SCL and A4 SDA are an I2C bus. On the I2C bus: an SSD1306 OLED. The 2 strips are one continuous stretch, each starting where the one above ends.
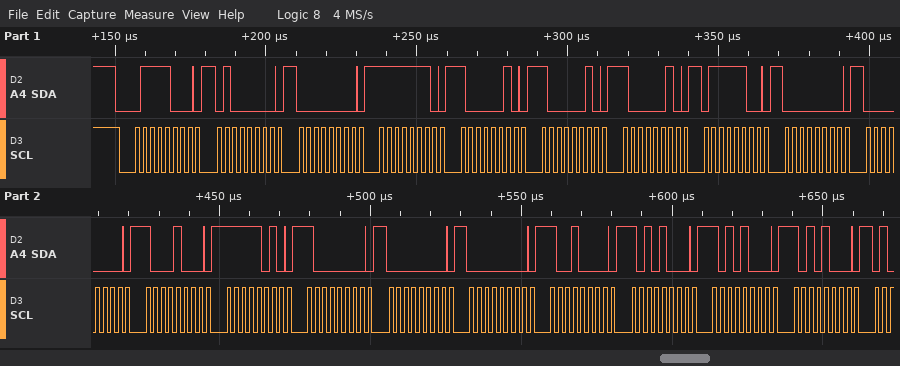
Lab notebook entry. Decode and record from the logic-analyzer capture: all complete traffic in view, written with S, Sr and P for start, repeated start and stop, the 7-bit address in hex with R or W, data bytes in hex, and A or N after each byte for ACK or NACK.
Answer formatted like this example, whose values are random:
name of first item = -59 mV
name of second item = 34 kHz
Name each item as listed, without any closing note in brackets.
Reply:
all complete traffic in view, written with S, Sr and P for start, repeated start and stop, the 7-bit address in hex with R or W, data bytes in hex, and A or N after each byte for ACK or NACK = S 3CW A 40 A 00 A FE A 82 A 82 A 82 A 7C A 00 A 00 A 88 A FA A 80 A 00 A 00 A 90 A A8 A A8 A A8 A
